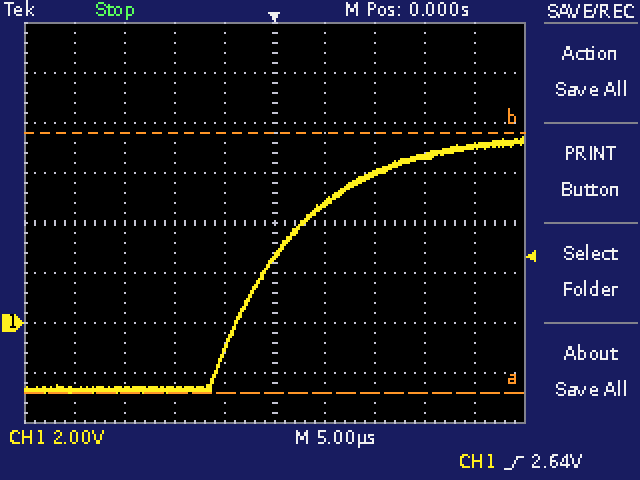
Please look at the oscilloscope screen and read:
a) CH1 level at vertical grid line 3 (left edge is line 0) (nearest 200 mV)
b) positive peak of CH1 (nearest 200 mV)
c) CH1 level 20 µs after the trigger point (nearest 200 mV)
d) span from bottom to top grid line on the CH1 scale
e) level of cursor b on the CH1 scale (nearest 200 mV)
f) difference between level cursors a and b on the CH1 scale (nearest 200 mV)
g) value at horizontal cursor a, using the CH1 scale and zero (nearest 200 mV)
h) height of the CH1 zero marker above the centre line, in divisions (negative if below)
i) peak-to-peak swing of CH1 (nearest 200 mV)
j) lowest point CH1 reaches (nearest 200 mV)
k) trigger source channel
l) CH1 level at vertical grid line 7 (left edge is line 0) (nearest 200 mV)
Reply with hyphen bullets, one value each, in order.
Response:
- -2.6 V
- 7.4 V
- 7.0 V
- 16 V
- 7.6 V
- 10.4 V
- -2.8 V
- -2.0 div
- 10.2 V
- -2.8 V
- CH1
- 6.0 V
